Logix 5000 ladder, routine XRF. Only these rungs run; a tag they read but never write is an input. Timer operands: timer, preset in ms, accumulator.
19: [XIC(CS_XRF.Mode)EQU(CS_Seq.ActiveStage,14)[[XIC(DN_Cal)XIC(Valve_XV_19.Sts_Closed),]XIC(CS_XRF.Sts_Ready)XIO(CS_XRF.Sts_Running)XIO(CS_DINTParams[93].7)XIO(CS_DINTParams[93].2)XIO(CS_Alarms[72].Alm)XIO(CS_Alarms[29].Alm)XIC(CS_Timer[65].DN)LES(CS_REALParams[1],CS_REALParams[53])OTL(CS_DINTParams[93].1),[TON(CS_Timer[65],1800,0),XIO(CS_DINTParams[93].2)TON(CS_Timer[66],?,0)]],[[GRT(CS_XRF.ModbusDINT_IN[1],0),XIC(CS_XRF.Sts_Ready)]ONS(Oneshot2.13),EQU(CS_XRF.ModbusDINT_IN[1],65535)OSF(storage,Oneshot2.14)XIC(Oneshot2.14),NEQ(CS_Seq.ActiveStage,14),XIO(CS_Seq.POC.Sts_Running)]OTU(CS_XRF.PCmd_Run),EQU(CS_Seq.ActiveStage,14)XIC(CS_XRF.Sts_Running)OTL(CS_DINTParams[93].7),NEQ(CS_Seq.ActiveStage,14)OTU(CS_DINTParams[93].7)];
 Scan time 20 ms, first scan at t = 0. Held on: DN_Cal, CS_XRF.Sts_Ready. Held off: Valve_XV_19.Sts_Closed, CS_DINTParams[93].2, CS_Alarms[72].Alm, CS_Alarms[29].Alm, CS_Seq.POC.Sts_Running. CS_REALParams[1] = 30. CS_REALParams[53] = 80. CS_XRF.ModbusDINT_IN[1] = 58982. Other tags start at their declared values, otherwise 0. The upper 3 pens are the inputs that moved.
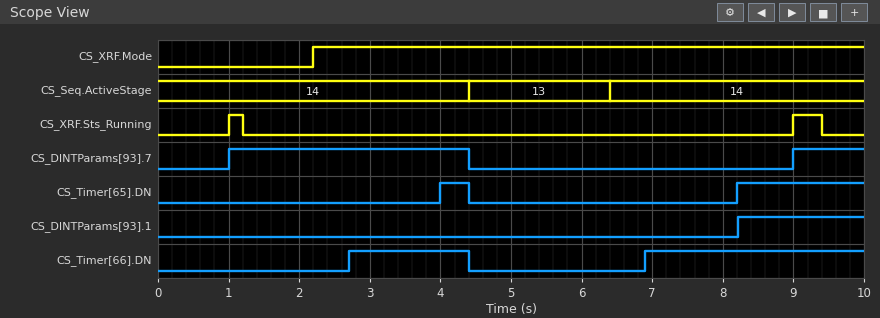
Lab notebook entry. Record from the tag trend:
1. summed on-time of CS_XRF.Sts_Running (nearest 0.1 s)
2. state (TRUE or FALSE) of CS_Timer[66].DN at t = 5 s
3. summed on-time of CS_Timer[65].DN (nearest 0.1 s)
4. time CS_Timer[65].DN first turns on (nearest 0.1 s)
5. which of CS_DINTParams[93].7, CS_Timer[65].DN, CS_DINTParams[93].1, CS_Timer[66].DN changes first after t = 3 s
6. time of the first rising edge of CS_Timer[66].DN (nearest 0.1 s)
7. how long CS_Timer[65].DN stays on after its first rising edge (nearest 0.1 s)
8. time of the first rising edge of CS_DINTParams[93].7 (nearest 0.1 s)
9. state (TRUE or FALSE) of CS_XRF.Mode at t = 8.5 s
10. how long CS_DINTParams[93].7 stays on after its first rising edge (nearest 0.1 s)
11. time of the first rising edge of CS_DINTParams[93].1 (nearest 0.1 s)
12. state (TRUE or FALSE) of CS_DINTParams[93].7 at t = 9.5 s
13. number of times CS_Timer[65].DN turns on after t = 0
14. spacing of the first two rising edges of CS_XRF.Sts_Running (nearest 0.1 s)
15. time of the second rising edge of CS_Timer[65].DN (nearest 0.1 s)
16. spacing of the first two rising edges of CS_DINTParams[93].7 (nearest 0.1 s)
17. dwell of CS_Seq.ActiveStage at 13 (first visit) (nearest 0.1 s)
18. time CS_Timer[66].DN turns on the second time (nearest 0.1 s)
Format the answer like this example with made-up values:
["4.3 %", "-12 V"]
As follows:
["0.6 s", "FALSE", "2.2 s", "4.0 s", "CS_Timer[65].DN", "2.7 s", "0.4 s", "1.0 s", "TRUE", "3.4 s", "8.2 s", "TRUE", "2", "8.0 s", "8.2 s", "8.0 s", "2.0 s", "6.9 s"]
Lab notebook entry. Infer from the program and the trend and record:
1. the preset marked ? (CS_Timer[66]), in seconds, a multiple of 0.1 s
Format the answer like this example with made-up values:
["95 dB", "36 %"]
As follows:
["0.5 s"]
